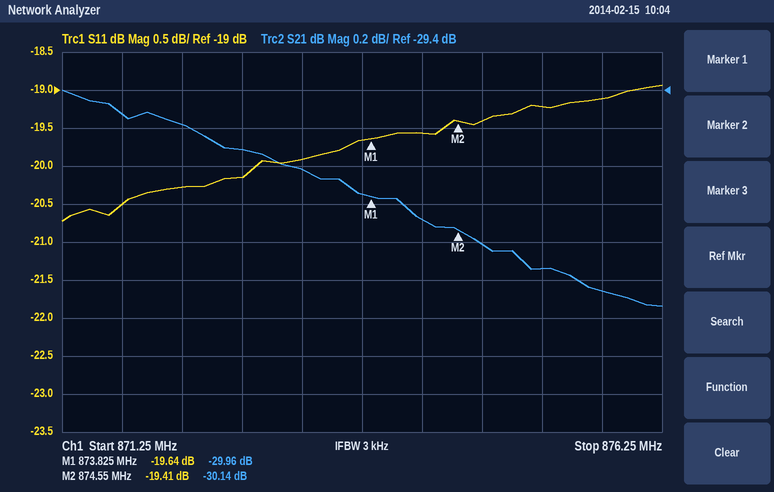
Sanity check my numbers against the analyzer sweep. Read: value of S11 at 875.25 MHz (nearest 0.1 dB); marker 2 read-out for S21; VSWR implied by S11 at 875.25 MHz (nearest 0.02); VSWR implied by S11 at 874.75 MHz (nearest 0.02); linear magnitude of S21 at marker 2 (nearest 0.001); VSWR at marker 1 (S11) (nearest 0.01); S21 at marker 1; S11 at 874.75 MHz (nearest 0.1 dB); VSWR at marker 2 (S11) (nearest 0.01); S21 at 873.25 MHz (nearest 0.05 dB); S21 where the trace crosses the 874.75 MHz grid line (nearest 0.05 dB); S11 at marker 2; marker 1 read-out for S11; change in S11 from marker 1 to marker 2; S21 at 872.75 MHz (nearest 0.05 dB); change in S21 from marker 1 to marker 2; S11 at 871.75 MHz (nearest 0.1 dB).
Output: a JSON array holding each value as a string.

["-19.2 dB", "-30.14 dB", "1.24", "1.24", "0.031", "1.23", "-29.96 dB", "-19.4 dB", "1.24", "-29.80 dB", "-30.20 dB", "-19.41 dB", "-19.64 dB", "0.23 dB", "-29.70 dB", "-0.18 dB", "-20.5 dB"]
